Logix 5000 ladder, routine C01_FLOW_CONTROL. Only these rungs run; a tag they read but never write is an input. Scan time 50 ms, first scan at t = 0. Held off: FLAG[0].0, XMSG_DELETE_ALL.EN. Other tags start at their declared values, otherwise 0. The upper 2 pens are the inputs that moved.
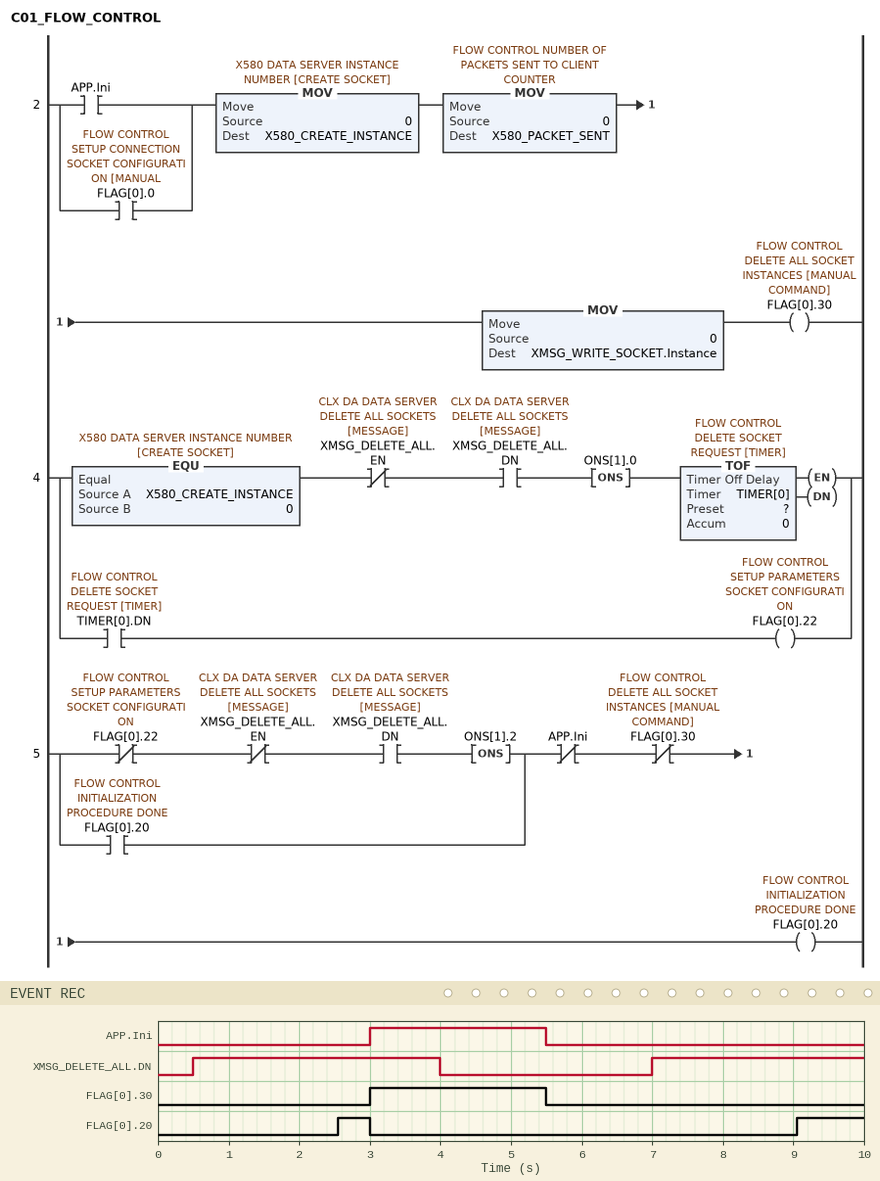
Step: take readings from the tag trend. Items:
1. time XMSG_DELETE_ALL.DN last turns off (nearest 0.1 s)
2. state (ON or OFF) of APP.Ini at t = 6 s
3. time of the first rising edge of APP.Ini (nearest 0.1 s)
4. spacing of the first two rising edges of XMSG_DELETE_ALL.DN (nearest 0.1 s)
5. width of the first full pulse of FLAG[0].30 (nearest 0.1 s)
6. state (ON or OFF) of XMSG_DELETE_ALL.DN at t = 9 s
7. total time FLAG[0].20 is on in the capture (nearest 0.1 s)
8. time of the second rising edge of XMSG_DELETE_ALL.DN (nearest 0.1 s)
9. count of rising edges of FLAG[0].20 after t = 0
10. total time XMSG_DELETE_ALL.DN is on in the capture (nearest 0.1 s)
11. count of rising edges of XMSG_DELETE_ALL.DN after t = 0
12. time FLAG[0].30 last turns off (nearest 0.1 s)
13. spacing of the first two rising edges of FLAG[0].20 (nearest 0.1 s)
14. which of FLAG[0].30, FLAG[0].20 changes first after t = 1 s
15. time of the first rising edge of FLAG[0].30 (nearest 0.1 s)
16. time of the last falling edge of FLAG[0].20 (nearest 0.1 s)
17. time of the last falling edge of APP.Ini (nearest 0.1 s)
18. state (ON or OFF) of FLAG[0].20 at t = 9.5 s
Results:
4.0 s
OFF
3.0 s
6.5 s
2.5 s
ON
1.4 s
7.0 s
2
6.5 s
2
5.5 s
6.5 s
FLAG[0].20
3.0 s
3.0 s
5.5 s
ON
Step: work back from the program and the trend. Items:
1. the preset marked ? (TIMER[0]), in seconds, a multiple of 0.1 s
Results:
2.0 s
